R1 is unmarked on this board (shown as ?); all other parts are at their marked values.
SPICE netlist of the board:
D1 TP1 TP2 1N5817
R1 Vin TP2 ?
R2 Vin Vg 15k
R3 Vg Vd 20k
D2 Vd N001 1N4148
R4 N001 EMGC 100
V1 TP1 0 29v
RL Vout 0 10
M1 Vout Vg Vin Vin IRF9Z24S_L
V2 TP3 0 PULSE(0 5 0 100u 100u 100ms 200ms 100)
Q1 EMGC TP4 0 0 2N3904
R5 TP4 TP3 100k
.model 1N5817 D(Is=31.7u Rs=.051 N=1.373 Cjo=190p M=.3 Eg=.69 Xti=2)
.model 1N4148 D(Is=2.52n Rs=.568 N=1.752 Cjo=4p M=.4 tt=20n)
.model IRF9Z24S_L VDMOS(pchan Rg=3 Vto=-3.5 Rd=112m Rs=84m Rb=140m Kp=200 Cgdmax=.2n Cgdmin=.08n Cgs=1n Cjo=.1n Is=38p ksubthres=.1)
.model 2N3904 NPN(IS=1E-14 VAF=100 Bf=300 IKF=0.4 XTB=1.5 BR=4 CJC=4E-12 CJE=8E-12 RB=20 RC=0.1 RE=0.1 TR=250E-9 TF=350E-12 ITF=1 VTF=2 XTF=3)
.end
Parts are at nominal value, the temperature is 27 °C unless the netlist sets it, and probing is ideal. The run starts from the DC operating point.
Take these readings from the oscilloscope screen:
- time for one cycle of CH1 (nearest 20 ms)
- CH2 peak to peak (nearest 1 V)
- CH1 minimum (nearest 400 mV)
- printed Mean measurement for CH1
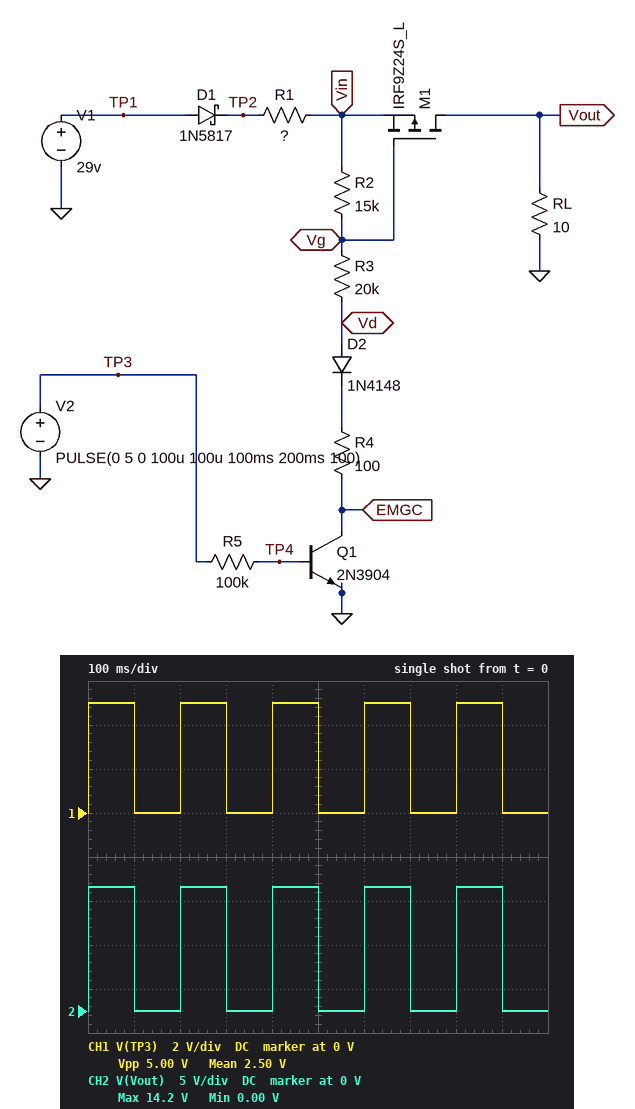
200 ms
14 V
0 V
2.50 V
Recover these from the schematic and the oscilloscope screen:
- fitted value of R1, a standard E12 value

10 Ω
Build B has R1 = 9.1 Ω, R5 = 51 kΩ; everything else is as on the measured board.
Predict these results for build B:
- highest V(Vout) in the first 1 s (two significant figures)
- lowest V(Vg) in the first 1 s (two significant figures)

15 V
8.9 V
